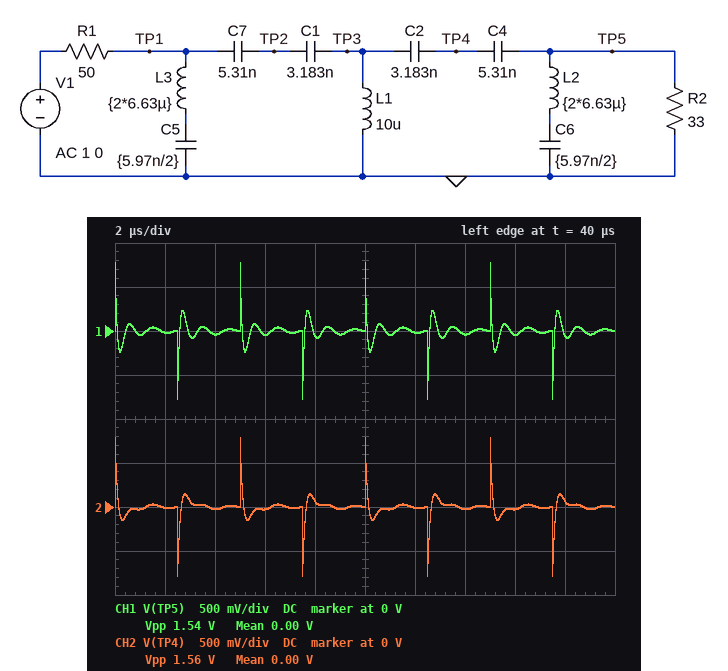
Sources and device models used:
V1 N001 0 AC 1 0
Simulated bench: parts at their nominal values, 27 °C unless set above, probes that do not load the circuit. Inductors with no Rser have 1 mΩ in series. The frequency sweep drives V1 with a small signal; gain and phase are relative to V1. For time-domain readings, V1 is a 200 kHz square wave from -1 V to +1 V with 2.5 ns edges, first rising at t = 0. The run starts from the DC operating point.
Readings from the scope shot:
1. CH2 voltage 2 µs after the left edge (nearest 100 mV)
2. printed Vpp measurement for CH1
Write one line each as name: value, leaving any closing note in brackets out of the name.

CH2 voltage 2 µs after the left edge: 0 V
printed Vpp measurement for CH1: 1.54 V
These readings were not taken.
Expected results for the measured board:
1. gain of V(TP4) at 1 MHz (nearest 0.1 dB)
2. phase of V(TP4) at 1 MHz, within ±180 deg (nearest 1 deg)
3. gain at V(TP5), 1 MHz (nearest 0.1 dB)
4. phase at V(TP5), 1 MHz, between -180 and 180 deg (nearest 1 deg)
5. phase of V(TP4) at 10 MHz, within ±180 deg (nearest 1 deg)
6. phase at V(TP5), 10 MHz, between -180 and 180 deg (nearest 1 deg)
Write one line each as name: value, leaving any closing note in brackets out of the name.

gain of V(TP4) at 1 MHz: -16.1 dB
phase of V(TP4) at 1 MHz, within ±180 deg: 106 deg
gain at V(TP5), 1 MHz: -15.2 dB
phase at V(TP5), 1 MHz, between -180 and 180 deg: -164 deg
phase of V(TP4) at 10 MHz, within ±180 deg: 10 deg
phase at V(TP5), 10 MHz, between -180 and 180 deg: 16 deg
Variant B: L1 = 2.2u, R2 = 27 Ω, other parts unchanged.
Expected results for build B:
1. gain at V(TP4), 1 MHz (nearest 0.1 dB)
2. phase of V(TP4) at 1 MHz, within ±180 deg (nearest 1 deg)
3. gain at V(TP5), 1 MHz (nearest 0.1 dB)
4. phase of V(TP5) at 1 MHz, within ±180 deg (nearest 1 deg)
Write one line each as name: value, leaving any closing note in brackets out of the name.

gain at V(TP4), 1 MHz: -23.5 dB
phase of V(TP4) at 1 MHz, within ±180 deg: -114 deg
gain at V(TP5), 1 MHz: -24.4 dB
phase of V(TP5) at 1 MHz, within ±180 deg: -24 deg
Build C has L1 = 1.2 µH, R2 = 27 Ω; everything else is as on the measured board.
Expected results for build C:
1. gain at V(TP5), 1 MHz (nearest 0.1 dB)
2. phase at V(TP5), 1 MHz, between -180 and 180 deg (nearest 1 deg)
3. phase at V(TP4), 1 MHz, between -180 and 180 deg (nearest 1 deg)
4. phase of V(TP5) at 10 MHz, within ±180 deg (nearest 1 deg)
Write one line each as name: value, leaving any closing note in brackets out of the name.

gain at V(TP5), 1 MHz: -32.1 dB
phase at V(TP5), 1 MHz, between -180 and 180 deg: -18 deg
phase at V(TP4), 1 MHz, between -180 and 180 deg: -108 deg
phase of V(TP5) at 10 MHz, within ±180 deg: 28 deg
